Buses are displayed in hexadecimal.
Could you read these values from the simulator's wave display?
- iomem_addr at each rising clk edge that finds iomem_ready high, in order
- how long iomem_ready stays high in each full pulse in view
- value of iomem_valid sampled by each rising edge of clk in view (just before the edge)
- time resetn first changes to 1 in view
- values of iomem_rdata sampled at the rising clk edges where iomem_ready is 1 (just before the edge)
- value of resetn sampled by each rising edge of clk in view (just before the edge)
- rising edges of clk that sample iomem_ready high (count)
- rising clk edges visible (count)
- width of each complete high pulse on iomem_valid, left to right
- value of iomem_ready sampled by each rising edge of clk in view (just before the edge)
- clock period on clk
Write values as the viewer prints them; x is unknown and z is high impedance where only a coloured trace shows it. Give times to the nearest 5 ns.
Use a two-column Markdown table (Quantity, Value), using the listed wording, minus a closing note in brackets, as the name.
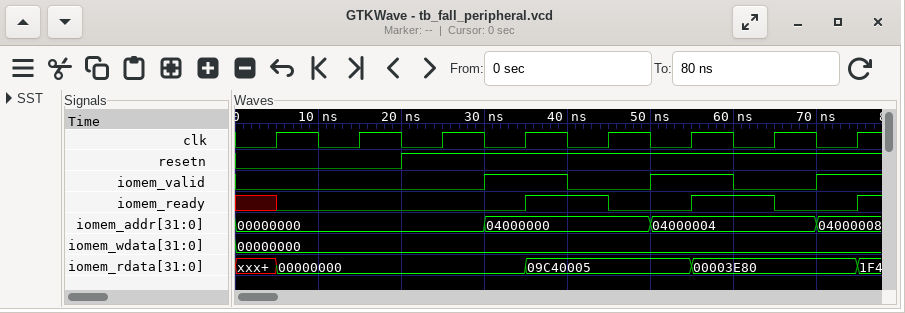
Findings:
| Quantity | Value |
|---|---|
| iomem_addr at each rising clk edge that finds iomem_ready high, in order | 04000000, 04000004 |
| how long iomem_ready stays high in each full pulse in view | 10 ns, 10 ns |
| value of iomem_valid sampled by each rising edge of clk in view | 0 0 0 1 0 1 0 1 |
| time resetn first changes to 1 in view | 20 ns |
| values of iomem_rdata sampled at the rising clk edges where iomem_ready is 1 | 09C40005, 00003E80 |
| value of resetn sampled by each rising edge of clk in view | 0 0 1 1 1 1 1 1 |
| rising edges of clk that sample iomem_ready high | 2 |
| rising clk edges visible | 8 |
| width of each complete high pulse on iomem_valid, left to right | 10 ns, 10 ns |
| value of iomem_ready sampled by each rising edge of clk in view | x 0 0 0 1 0 1 0 |
| clock period on clk | 10 ns |
